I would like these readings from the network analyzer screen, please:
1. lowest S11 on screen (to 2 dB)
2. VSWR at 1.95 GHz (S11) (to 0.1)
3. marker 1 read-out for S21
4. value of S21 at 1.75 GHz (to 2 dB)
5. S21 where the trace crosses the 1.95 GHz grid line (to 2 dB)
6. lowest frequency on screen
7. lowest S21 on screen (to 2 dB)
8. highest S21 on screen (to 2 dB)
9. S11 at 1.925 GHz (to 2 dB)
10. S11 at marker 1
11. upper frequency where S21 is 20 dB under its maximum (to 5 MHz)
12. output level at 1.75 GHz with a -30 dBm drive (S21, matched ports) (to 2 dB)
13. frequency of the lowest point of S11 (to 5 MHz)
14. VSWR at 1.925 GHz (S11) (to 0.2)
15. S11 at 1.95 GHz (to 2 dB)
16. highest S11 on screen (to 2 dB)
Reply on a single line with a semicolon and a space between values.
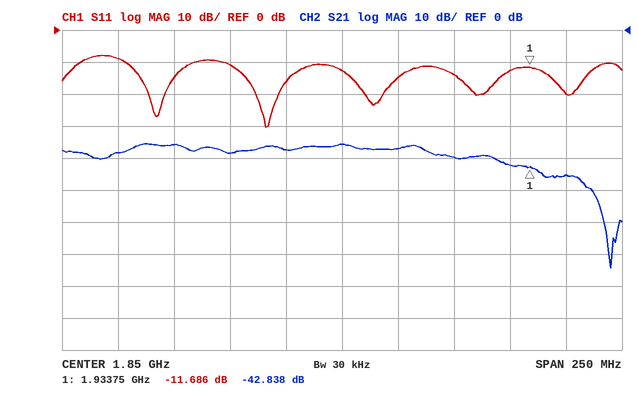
-30 dB; 1.2; -42.838 dB; -38 dB; -46 dB; 1.725 GHz; -74 dB; -36 dB; -12 dB; -11.686 dB; 1.965 GHz; -68 dBm; 1.815 GHz; 1.6; -20 dB; -8 dB
